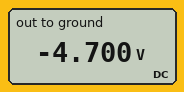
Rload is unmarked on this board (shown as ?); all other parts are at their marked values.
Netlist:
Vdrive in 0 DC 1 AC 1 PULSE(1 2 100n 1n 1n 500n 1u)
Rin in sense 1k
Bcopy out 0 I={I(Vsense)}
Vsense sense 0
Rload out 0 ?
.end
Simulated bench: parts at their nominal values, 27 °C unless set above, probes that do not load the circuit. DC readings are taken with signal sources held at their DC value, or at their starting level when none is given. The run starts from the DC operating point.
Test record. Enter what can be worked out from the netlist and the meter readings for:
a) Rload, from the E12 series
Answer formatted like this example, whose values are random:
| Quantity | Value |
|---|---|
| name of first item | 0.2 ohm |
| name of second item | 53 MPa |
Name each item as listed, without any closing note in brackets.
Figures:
| Quantity | Value |
|---|---|
| Rload, from the E12 series | 4.7 kΩ |
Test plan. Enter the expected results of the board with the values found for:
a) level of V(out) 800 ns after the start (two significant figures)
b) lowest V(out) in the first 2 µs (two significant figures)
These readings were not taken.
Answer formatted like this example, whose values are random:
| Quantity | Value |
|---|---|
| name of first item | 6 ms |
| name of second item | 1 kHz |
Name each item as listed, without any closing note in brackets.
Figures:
| Quantity | Value |
|---|---|
| level of V(out) 800 ns after the start | -4.7 V |
| lowest V(out) in the first 2 µs | -9.4 V |
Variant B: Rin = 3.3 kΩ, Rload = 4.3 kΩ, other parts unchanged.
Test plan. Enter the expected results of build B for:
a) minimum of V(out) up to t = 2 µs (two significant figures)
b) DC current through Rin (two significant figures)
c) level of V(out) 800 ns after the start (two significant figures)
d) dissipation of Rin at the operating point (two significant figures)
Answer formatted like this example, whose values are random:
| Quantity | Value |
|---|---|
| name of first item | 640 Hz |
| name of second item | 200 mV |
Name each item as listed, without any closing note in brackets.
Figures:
| Quantity | Value |
|---|---|
| minimum of V(out) up to t = 2 µs | -2.6 V |
| DC current through Rin | 300 µA |
| level of V(out) 800 ns after the start | -1.3 V |
| dissipation of Rin at the operating point | 300 µW |
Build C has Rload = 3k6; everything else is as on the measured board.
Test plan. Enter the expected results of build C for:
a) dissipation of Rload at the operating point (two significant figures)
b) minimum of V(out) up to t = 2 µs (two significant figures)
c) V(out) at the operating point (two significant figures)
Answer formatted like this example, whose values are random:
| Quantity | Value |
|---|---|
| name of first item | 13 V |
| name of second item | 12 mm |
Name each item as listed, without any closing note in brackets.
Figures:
| Quantity | Value |
|---|---|
| dissipation of Rload at the operating point | 3.6 mW |
| minimum of V(out) up to t = 2 µs | -7.2 V |
| V(out) at the operating point | -3.6 V |
